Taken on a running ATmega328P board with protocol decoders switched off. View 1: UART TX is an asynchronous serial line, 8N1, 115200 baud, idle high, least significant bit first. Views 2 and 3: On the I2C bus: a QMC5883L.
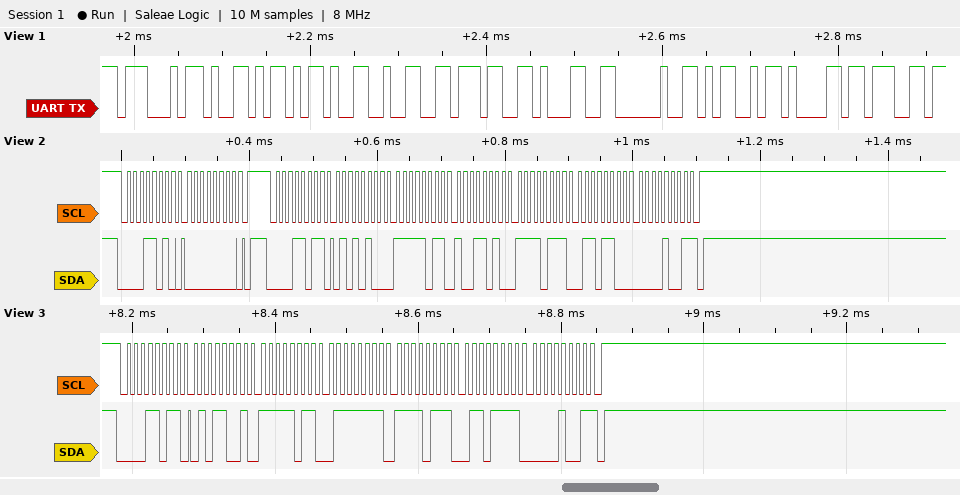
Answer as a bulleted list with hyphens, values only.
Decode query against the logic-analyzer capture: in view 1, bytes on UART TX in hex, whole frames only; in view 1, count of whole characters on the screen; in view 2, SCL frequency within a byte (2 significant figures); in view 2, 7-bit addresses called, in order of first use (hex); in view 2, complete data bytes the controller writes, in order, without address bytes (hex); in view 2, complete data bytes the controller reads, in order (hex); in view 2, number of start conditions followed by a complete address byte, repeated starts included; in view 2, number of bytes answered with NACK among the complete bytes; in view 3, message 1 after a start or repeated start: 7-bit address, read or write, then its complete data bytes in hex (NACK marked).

- 47 59 2D 32 37 31 20 4D 61 67
- 10
- 100 kHz
- 0x0D
- 00
- 54 FB 9A F7 6C 09
- 2
- 1
- 0x0D read: 59 FB 7F F7 6F 09 NACK
